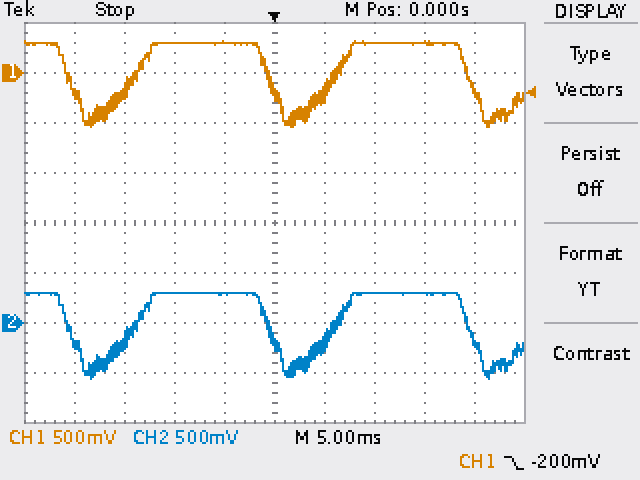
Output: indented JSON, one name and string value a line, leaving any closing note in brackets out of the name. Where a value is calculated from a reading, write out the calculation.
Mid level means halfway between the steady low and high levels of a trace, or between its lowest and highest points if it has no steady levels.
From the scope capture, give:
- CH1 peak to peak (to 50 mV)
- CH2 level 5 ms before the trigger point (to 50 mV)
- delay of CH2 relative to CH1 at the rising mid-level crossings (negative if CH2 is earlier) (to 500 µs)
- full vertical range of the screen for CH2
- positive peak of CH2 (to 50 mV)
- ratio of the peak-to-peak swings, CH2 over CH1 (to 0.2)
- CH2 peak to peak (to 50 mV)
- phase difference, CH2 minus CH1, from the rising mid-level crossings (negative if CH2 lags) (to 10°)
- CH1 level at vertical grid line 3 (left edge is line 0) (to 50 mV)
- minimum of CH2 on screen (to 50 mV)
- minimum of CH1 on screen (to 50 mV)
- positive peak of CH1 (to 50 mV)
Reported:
{
  "CH1 peak to peak": "300 mV − (-550 mV) = 850 mV",
  "CH2 level 5 ms before the trigger point": "300 mV",
  "delay of CH2 relative to CH1 at the rising mid-level crossings (negative if CH2 is earlier)": "0.0 ms",
  "full vertical range of the screen for CH2": "4 V",
  "positive peak of CH2": "300 mV",
  "ratio of the peak-to-peak swings, CH2 over CH1": "850 mV / 850 mV ≈ 1.0",
  "CH2 peak to peak": "300 mV − (-550 mV) = 850 mV",
  "phase difference, CH2 minus CH1, from the rising mid-level crossings (negative if CH2 lags)": "0°",
  "CH1 level at vertical grid line 3 (left edge is line 0)": "300 mV",
  "minimum of CH2 on screen": "-550 mV",
  "minimum of CH1 on screen": "-550 mV",
  "positive peak of CH1": "300 mV"
}
